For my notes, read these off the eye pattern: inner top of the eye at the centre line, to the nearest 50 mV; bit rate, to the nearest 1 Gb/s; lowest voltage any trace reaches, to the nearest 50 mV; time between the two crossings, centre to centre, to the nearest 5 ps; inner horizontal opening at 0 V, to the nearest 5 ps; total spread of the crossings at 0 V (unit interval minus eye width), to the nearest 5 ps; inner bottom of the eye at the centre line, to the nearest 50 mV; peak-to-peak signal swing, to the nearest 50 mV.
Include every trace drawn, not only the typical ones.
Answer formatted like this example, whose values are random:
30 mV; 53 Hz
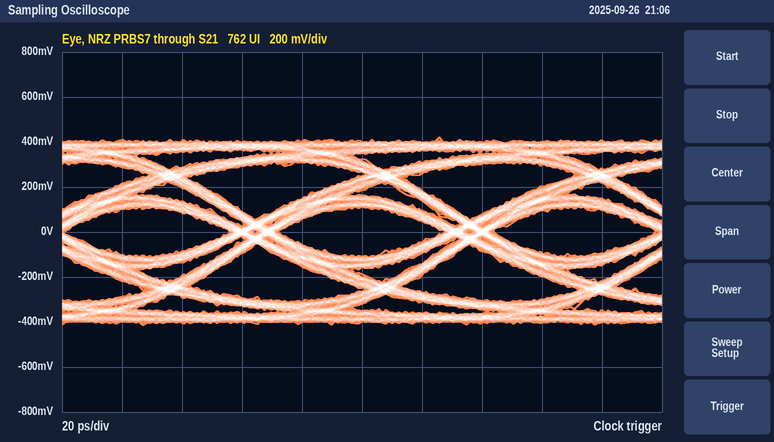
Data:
100 mV; 14 Gb/s; -400 mV; 70 ps; 55 ps; 15 ps; -100 mV; 850 mV
